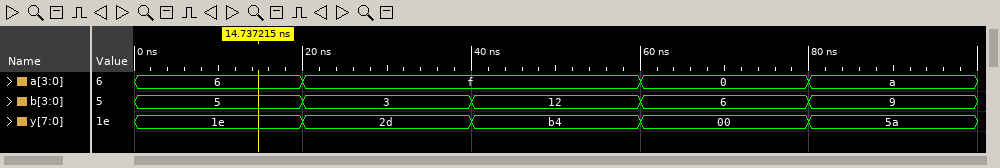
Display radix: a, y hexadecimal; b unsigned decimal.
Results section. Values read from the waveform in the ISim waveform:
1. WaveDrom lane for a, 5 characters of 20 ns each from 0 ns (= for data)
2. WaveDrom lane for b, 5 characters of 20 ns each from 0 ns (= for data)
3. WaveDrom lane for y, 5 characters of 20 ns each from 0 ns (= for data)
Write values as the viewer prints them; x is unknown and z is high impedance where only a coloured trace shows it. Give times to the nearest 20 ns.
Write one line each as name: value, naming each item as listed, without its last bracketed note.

WaveDrom lane for a, 5 characters of 20 ns each from 0 ns: {name: 'a', wave: '==.==', data: '6 f 0 a'}
WaveDrom lane for b, 5 characters of 20 ns each from 0 ns: {name: 'b', wave: '=====', data: '5 3 12 6 9'}
WaveDrom lane for y, 5 characters of 20 ns each from 0 ns: {name: 'y', wave: '=====', data: '1e 2d b4 00 5a'}
